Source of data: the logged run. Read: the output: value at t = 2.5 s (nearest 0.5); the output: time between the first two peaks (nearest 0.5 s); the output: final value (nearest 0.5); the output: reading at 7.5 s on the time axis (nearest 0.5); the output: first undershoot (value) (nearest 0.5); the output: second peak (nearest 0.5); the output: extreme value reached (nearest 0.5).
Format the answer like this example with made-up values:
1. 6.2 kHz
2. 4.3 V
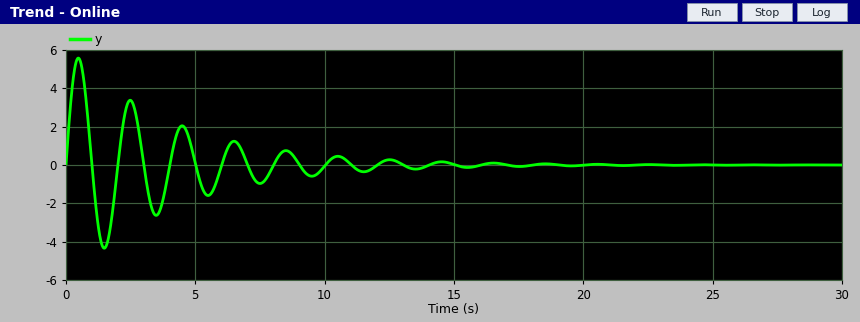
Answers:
1. 3.5
2. 2.0 s
3. 0.0
4. -1.0
5. -4.5
6. 3.5
7. 5.5
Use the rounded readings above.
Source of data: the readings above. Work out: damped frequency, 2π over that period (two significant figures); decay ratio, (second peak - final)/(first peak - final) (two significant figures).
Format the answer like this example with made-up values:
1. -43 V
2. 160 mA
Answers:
1. 3.1 rad/s
2. 0.64
